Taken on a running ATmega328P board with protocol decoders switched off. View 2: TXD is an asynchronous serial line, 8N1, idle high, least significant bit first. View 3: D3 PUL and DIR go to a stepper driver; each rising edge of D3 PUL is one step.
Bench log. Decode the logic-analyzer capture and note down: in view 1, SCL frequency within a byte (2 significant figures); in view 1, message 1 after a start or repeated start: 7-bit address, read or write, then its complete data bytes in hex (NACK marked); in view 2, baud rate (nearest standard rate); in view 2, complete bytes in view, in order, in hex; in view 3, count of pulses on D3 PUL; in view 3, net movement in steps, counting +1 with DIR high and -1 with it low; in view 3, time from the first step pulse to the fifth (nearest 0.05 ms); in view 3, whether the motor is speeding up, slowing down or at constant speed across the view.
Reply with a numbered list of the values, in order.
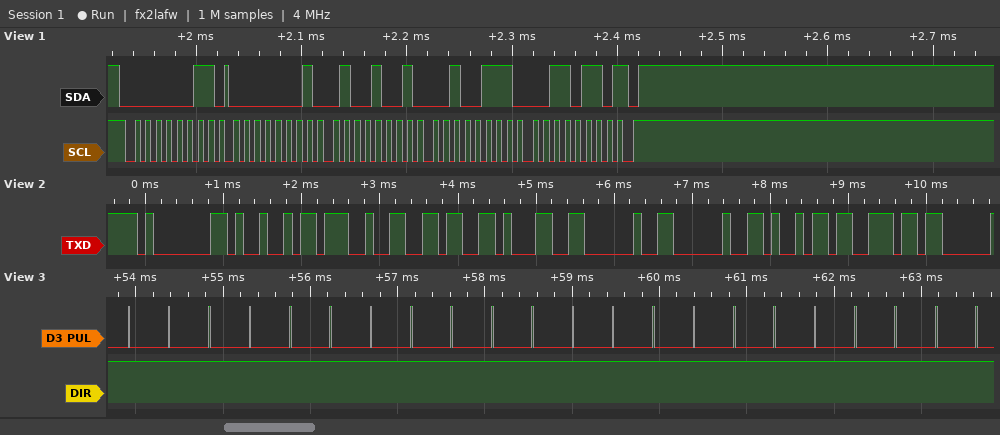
1. 100 kHz
2. 0x01 read: 01 49 27 36 NACK
3. 9600 baud
4. 01 49 27 36 31 20 20 69 6E
5. 22
6. +22
7. 1.85 ms
8. constant speed
